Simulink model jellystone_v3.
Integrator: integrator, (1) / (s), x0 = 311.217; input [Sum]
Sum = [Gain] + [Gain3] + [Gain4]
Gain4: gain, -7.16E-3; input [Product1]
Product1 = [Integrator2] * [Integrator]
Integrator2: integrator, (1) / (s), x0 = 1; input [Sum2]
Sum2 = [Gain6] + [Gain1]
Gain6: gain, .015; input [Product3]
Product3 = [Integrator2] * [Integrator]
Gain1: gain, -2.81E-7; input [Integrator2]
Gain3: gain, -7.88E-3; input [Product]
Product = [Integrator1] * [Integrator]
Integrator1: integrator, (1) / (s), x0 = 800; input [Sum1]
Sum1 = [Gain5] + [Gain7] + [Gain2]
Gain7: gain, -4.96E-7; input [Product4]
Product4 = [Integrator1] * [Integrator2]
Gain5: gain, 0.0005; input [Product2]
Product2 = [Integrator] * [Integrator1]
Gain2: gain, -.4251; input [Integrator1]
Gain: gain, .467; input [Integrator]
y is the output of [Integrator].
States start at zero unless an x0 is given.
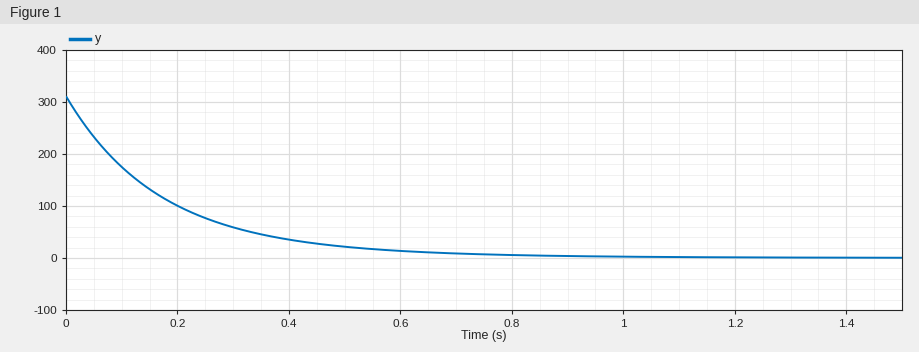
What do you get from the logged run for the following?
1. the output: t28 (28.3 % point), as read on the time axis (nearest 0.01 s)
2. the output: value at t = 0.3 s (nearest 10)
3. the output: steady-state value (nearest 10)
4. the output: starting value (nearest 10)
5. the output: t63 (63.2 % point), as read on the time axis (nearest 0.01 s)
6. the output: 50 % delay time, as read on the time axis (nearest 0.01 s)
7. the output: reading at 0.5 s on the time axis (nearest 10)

0.06 s
60
0
310
0.18 s
0.12 s
20
